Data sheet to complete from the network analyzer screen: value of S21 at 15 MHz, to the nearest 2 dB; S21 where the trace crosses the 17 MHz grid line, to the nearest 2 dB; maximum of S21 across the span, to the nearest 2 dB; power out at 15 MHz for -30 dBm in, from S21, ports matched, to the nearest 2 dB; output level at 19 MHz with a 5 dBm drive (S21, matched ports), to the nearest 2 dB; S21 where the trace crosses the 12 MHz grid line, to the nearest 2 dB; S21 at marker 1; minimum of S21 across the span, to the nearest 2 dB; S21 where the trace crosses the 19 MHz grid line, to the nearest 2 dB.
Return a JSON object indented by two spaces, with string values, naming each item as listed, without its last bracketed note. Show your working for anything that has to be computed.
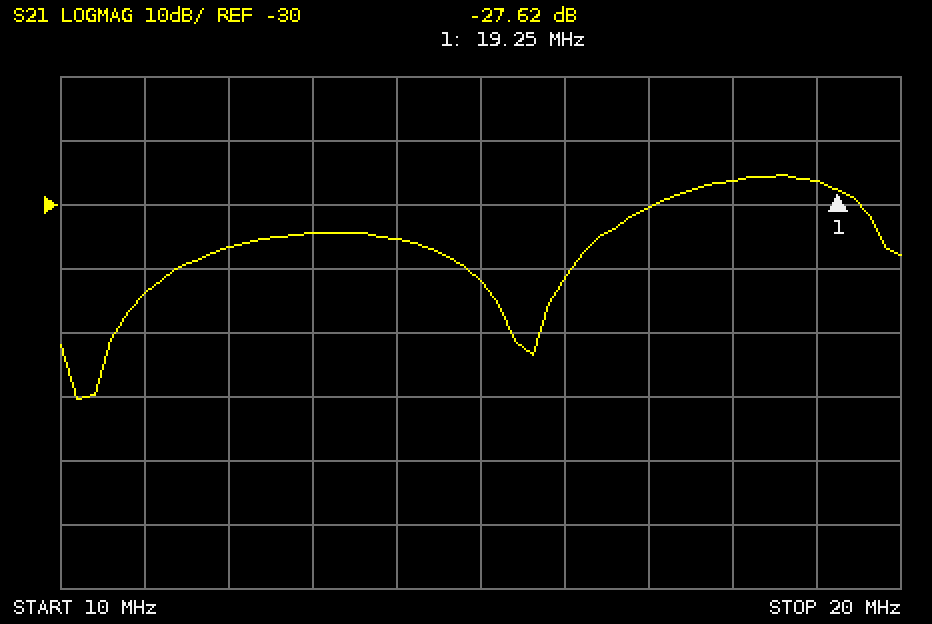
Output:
{
  "value of S21 at 15 MHz, to the nearest 2 dB": "-42 dB",
  "S21 where the trace crosses the 17 MHz grid line, to the nearest 2 dB": "-30 dB",
  "maximum of S21 across the span, to the nearest 2 dB": "-26 dB",
  "power out at 15 MHz for -30 dBm in, from S21, ports matched, to the nearest 2 dB": "-30 dBm + (-42 dB) = -72 dBm",
  "output level at 19 MHz with a 5 dBm drive (S21, matched ports), to the nearest 2 dB": "5 dBm + (-26 dB) = -22 dBm",
  "S21 where the trace crosses the 12 MHz grid line, to the nearest 2 dB": "-36 dB",
  "S21 at marker 1": "-27.62 dB",
  "minimum of S21 across the span, to the nearest 2 dB": "-60 dB",
  "S21 where the trace crosses the 19 MHz grid line, to the nearest 2 dB": "-26 dB"
}
